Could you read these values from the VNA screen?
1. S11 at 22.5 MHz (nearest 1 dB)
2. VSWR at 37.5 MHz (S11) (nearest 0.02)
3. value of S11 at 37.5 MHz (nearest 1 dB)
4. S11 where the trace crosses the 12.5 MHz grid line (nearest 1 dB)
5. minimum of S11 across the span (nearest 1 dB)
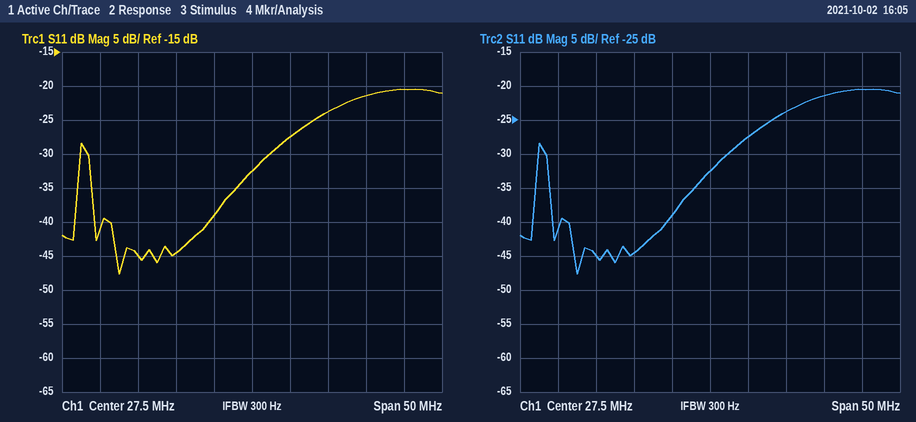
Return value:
-39 dB
1.14
-24 dB
-45 dB
-48 dB
